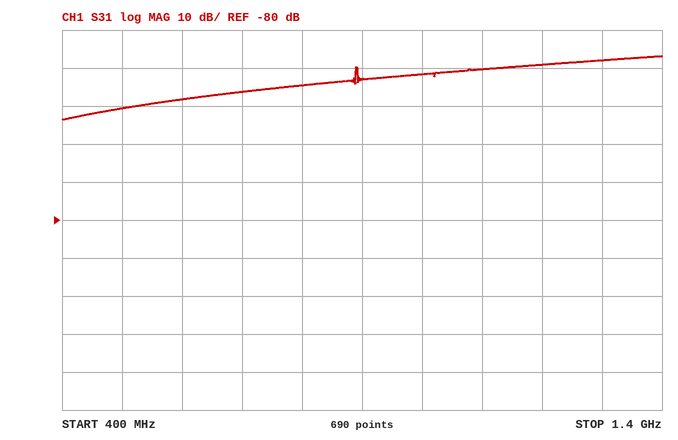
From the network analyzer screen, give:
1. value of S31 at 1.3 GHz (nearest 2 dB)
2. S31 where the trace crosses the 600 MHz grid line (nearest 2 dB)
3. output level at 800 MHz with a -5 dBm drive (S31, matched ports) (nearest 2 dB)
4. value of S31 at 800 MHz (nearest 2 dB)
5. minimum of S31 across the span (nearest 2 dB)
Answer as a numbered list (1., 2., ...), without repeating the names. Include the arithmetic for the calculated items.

1. -38 dB
2. -48 dB
3. -5 dBm + (-44 dB) = -50 dBm
4. -44 dB
5. -54 dB
